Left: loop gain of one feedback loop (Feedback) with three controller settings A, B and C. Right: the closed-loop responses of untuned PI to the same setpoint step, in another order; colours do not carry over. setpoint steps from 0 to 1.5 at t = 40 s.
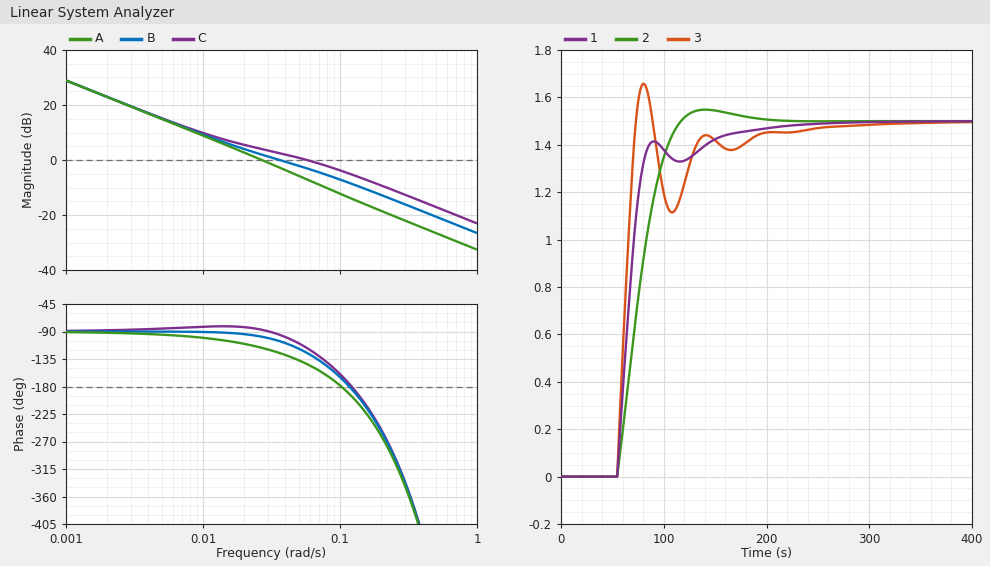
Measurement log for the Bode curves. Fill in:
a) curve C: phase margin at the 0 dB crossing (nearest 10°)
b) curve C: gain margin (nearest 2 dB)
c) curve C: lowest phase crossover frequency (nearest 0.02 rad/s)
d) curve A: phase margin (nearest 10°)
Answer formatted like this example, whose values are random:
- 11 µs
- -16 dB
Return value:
- 60°
- 6 dB
- 0.12 rad/s
- 60°
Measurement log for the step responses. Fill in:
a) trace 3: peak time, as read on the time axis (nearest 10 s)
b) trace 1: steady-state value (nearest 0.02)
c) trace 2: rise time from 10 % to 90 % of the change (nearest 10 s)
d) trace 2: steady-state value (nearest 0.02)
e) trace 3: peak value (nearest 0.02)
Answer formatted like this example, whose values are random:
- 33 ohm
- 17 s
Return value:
- 80 s
- 1.50
- 40 s
- 1.50
- 1.66
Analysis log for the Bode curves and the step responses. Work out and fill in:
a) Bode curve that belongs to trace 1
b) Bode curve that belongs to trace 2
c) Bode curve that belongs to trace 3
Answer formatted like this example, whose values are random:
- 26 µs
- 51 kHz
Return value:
- B
- A
- C
